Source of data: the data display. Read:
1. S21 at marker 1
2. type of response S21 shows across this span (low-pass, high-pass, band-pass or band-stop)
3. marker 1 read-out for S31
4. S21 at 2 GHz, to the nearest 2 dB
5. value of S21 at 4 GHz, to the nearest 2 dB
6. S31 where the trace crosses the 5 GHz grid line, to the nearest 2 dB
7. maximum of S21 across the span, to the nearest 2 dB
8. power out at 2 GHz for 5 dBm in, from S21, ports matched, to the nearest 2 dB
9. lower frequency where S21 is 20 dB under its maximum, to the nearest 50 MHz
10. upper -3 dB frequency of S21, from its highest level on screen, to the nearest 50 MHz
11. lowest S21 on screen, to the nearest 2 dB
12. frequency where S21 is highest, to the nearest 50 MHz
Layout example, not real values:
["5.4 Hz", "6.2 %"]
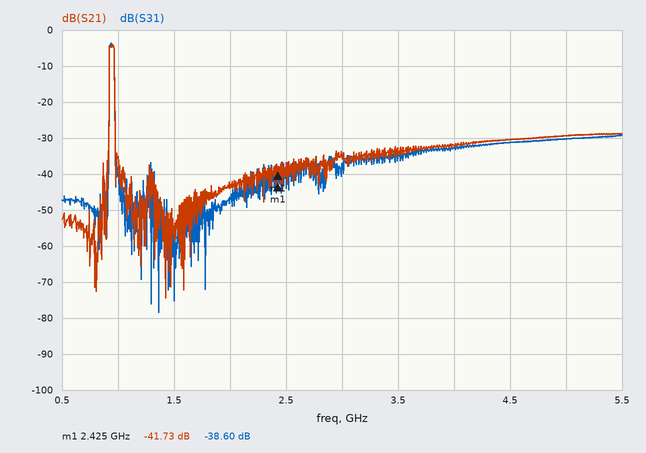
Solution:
["-41.73 dB", "band-pass", "-38.60 dB", "-44 dB", "-32 dB", "-30 dB", "-4 dB", "-38 dBm", "900 MHz", "950 MHz", "-74 dB", "950 MHz"]
